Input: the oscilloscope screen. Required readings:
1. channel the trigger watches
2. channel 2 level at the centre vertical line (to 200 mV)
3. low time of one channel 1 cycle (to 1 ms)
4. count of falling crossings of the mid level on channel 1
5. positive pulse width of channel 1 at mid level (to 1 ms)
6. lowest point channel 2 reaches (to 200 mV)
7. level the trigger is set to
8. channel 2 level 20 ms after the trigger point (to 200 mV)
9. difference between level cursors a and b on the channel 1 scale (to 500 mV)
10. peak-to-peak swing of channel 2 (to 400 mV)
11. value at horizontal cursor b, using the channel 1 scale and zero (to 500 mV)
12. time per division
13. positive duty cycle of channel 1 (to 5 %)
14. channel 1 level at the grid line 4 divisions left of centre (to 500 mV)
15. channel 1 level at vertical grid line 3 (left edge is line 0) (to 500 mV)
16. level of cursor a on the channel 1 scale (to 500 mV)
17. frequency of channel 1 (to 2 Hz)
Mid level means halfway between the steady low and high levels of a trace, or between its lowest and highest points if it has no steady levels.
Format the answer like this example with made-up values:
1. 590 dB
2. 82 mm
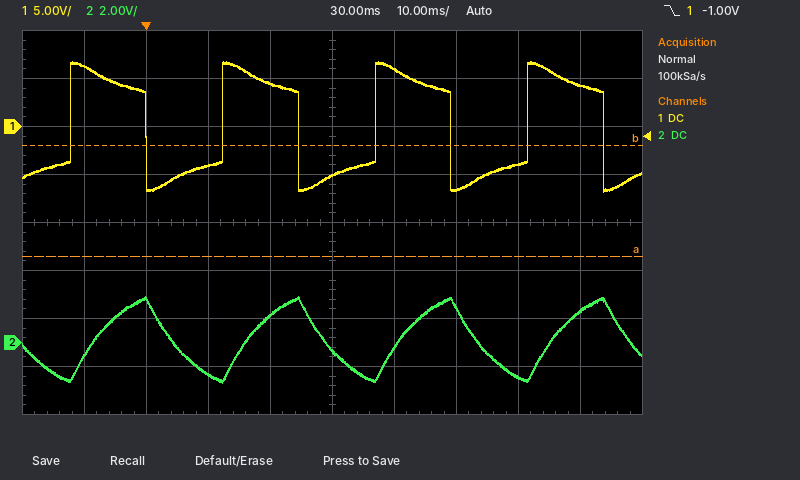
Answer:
1. channel 1
2. -400 mV
3. 12 ms
4. 4
5. 12 ms
6. -1.6 V
7. -1.00 V
8. 1.2 V
9. 11.5 V
10. 3.6 V
11. -2.0 V
12. 10 ms
13. 50 %
14. 6.5 V
15. -4.0 V
16. -13.5 V
17. 40 Hz
